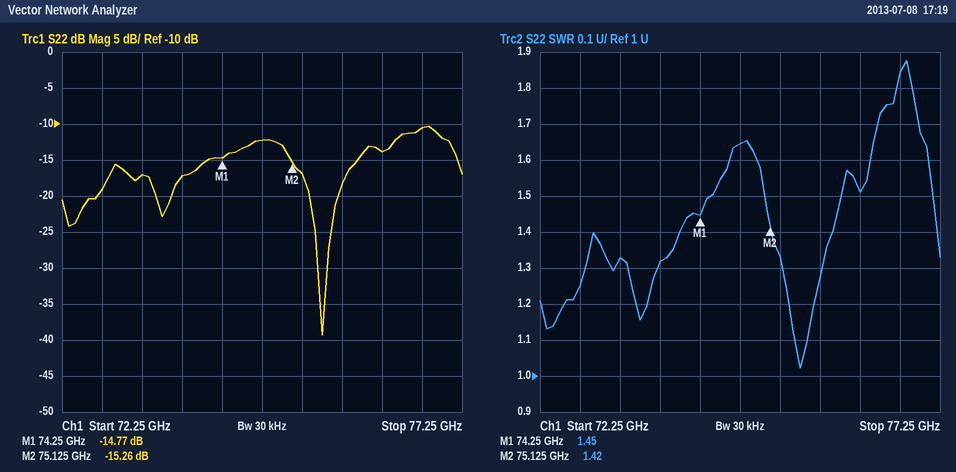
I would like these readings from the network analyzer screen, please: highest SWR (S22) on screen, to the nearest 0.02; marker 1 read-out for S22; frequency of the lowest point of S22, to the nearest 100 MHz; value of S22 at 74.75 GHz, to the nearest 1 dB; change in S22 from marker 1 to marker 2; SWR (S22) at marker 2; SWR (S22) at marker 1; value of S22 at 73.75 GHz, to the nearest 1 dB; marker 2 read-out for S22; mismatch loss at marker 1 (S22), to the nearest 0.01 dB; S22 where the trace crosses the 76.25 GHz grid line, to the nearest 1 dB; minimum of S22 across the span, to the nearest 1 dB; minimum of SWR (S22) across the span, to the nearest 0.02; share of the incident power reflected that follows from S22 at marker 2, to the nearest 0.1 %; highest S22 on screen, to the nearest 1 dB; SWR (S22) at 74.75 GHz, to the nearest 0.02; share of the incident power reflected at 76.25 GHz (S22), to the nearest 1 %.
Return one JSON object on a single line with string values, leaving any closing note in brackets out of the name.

{"highest SWR (S22) on screen, to the nearest 0.02": "1.88", "marker 1 read-out for S22": "-14.77 dB", "frequency of the lowest point of S22, to the nearest 100 MHz": "75.5 GHz", "value of S22 at 74.75 GHz, to the nearest 1 dB": "-12 dB", "change in S22 from marker 1 to marker 2": "-0.49 dB", "SWR (S22) at marker 2": "1.42", "SWR (S22) at marker 1": "1.45", "value of S22 at 73.75 GHz, to the nearest 1 dB": "-17 dB", "marker 2 read-out for S22": "-15.26 dB", "mismatch loss at marker 1 (S22), to the nearest 0.01 dB": "0.15 dB", "S22 where the trace crosses the 76.25 GHz grid line, to the nearest 1 dB": "-14 dB", "minimum of S22 across the span, to the nearest 1 dB": "-39 dB", "minimum of SWR (S22) across the span, to the nearest 0.02": "1.02", "share of the incident power reflected that follows from S22 at marker 2, to the nearest 0.1 %": "3.0 %", "highest S22 on screen, to the nearest 1 dB": "-10 dB", "SWR (S22) at 74.75 GHz, to the nearest 0.02": "1.64", "share of the incident power reflected at 76.25 GHz (S22), to the nearest 1 %": "4 %"}
